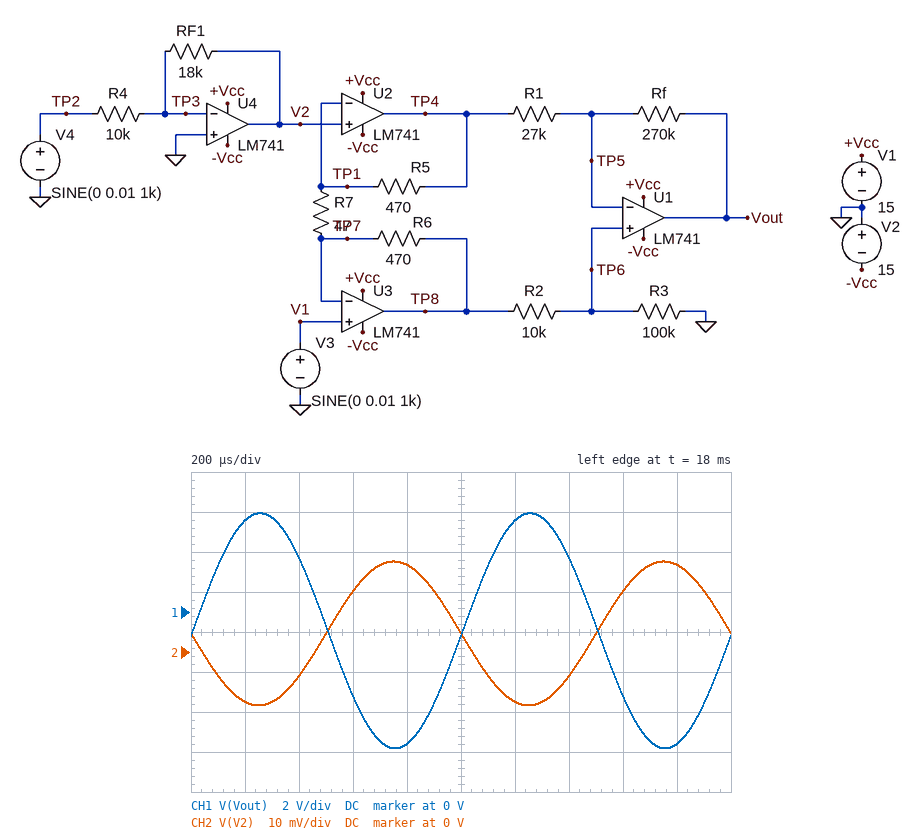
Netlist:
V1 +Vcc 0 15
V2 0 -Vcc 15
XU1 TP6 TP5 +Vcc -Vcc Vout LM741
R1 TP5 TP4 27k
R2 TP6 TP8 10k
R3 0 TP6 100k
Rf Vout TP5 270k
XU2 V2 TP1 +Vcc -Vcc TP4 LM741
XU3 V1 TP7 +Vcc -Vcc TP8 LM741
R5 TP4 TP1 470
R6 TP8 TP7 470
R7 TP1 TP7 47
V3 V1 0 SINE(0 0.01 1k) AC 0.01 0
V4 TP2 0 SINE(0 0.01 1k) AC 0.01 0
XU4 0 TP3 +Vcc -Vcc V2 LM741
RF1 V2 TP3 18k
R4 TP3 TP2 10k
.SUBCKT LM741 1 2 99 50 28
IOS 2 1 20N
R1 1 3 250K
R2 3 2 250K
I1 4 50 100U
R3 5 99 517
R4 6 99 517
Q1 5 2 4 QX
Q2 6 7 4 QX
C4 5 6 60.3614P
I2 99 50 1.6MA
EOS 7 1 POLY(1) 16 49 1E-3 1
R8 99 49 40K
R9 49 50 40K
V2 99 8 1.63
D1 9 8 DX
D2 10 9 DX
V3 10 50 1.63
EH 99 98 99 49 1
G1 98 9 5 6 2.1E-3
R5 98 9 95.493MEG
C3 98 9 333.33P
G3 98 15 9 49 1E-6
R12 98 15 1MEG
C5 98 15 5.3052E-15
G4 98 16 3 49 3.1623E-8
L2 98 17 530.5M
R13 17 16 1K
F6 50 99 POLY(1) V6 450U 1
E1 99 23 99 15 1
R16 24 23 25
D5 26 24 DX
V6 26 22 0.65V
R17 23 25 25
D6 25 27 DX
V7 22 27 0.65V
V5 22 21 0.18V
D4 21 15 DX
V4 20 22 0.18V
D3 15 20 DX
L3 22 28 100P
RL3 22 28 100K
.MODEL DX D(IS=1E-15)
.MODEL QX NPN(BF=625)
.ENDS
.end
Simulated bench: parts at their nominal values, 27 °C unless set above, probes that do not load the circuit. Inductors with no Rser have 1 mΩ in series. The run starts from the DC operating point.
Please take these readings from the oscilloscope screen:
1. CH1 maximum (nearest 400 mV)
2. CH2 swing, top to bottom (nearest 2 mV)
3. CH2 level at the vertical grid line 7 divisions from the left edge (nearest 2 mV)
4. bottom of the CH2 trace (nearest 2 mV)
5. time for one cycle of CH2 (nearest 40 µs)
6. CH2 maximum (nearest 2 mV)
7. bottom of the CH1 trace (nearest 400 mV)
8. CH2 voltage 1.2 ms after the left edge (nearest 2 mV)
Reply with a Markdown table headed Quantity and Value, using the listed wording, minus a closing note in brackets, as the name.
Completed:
| Quantity | Value |
|---|---|
| CH1 maximum | 4.8 V |
| CH2 swing, top to bottom | 36 mV |
| CH2 level at the vertical grid line 7 divisions from the left edge | -6 mV |
| bottom of the CH2 trace | -14 mV |
| time for one cycle of CH2 | 1.00 ms |
| CH2 maximum | 22 mV |
| bottom of the CH1 trace | -6.8 V |
| CH2 voltage 1.2 ms after the left edge | -12 mV |
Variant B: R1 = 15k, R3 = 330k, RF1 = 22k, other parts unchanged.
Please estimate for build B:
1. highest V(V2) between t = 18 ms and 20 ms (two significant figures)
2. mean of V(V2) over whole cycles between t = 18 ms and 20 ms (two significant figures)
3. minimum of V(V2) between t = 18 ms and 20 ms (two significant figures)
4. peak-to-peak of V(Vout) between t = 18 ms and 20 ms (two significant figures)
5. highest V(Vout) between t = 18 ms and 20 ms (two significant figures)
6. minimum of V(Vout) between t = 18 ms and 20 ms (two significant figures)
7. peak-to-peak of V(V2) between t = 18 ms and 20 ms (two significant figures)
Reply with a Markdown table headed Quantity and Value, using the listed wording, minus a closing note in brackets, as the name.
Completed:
| Quantity | Value |
|---|---|
| highest V(V2) between t = 18 ms and 20 ms | 27 mV |
| mean of V(V2) over whole cycles between t = 18 ms and 20 ms | 5.4 mV |
| minimum of V(V2) between t = 18 ms and 20 ms | -17 mV |
| peak-to-peak of V(Vout) between t = 18 ms and 20 ms | 24 V |
| highest V(Vout) between t = 18 ms and 20 ms | 10 V |
| minimum of V(Vout) between t = 18 ms and 20 ms | -14 V |
| peak-to-peak of V(V2) between t = 18 ms and 20 ms | 44 mV |
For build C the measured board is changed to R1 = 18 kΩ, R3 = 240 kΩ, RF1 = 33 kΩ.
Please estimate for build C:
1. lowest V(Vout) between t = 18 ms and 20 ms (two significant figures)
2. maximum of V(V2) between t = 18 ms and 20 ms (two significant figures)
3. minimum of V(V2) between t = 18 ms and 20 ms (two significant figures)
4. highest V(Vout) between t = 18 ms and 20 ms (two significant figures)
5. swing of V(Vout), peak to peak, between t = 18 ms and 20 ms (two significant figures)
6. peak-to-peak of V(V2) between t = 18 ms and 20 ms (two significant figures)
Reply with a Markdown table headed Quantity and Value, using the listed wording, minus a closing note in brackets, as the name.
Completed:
| Quantity | Value |
|---|---|
| lowest V(Vout) between t = 18 ms and 20 ms | -14 V |
| maximum of V(V2) between t = 18 ms and 20 ms | 41 mV |
| minimum of V(V2) between t = 18 ms and 20 ms | -25 mV |
| highest V(Vout) between t = 18 ms and 20 ms | 11 V |
| swing of V(Vout), peak to peak, between t = 18 ms and 20 ms | 25 V |
| peak-to-peak of V(V2) between t = 18 ms and 20 ms | 66 mV |
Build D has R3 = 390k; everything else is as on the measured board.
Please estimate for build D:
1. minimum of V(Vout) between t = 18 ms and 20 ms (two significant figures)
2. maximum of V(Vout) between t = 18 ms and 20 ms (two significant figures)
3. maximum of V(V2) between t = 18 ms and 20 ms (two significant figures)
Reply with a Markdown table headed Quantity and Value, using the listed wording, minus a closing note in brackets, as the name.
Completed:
| Quantity | Value |
|---|---|
| minimum of V(Vout) between t = 18 ms and 20 ms | -7.1 V |
| maximum of V(Vout) between t = 18 ms and 20 ms | 5.1 V |
| maximum of V(V2) between t = 18 ms and 20 ms | 23 mV |
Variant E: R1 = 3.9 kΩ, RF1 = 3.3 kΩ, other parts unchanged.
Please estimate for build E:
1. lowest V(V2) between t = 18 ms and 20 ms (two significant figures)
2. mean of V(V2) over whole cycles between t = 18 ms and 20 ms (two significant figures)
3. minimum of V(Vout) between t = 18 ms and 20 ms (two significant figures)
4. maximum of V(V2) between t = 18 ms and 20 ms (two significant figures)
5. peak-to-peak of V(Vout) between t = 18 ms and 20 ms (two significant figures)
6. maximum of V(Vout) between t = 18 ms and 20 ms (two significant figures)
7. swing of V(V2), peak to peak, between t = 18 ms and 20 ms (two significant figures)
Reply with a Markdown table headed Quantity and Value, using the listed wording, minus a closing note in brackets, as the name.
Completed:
| Quantity | Value |
|---|---|
| lowest V(V2) between t = 18 ms and 20 ms | -1.6 mV |
| mean of V(V2) over whole cycles between t = 18 ms and 20 ms | 1.7 mV |
| minimum of V(Vout) between t = 18 ms and 20 ms | -14 V |
| maximum of V(V2) between t = 18 ms and 20 ms | 5.0 mV |
| peak-to-peak of V(Vout) between t = 18 ms and 20 ms | 28 V |
| maximum of V(Vout) between t = 18 ms and 20 ms | 14 V |
| swing of V(V2), peak to peak, between t = 18 ms and 20 ms | 6.6 mV |
